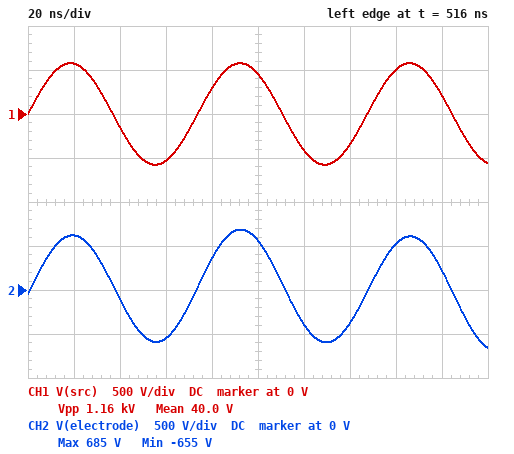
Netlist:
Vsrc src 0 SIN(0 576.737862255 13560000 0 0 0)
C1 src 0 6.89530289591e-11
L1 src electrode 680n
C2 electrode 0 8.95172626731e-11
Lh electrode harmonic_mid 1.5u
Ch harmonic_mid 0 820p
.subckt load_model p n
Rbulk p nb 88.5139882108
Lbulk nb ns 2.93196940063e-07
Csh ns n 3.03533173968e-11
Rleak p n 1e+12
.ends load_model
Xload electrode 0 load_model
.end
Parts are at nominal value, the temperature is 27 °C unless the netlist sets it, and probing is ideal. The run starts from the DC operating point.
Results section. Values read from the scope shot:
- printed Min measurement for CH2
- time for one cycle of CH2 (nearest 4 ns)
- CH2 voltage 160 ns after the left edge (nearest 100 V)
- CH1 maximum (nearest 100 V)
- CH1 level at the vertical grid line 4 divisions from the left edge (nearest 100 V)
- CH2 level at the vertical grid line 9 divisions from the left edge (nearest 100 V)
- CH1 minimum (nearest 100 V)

-655 V
76 ns
500 V
600 V
300 V
200 V
-600 V
